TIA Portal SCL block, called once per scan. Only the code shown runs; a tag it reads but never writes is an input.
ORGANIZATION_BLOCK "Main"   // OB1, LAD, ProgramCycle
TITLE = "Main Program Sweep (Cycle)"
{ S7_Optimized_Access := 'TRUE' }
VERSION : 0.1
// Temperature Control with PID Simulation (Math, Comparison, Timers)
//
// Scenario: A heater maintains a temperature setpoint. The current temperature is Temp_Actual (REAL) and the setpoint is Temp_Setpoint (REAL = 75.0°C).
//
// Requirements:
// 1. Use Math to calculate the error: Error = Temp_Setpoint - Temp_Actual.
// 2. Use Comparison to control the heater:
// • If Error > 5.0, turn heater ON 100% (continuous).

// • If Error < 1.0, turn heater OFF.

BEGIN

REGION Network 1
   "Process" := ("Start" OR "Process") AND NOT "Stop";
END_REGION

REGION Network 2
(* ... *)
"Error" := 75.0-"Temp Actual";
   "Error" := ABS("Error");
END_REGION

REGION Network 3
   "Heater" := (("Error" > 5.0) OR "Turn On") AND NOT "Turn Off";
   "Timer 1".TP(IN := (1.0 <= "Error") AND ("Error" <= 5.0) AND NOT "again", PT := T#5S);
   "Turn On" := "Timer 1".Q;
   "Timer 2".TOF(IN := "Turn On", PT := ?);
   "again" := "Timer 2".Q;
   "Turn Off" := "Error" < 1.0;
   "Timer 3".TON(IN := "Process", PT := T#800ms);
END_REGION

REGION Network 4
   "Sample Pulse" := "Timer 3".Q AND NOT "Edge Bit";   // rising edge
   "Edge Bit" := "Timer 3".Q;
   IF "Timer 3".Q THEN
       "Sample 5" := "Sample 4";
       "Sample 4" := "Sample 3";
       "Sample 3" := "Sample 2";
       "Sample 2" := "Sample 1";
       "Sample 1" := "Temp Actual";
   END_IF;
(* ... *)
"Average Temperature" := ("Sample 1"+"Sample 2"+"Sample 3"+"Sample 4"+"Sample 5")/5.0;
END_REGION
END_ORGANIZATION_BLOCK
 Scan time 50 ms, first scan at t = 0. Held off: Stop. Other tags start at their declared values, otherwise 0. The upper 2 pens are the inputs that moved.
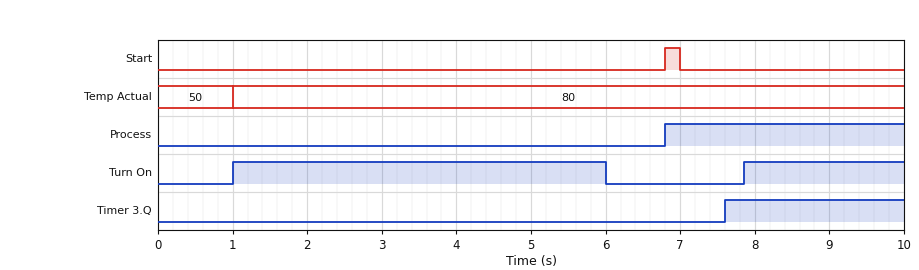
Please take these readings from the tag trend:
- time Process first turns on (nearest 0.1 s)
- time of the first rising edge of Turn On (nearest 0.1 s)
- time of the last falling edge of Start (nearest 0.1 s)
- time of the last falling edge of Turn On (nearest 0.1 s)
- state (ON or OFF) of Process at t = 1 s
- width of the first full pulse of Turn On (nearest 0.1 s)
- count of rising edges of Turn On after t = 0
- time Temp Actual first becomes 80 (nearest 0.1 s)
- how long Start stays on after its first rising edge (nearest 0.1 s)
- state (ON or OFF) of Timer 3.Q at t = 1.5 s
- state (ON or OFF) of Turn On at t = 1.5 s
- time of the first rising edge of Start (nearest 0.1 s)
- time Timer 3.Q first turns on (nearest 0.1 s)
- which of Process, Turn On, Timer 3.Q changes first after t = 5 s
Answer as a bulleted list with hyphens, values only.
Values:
- 6.8 s
- 1.0 s
- 7.0 s
- 6.0 s
- OFF
- 5.0 s
- 2
- 1.0 s
- 0.2 s
- OFF
- ON
- 6.8 s
- 7.6 s
- Turn On
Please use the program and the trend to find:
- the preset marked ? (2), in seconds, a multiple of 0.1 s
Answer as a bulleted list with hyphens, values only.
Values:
- 1.8 s
